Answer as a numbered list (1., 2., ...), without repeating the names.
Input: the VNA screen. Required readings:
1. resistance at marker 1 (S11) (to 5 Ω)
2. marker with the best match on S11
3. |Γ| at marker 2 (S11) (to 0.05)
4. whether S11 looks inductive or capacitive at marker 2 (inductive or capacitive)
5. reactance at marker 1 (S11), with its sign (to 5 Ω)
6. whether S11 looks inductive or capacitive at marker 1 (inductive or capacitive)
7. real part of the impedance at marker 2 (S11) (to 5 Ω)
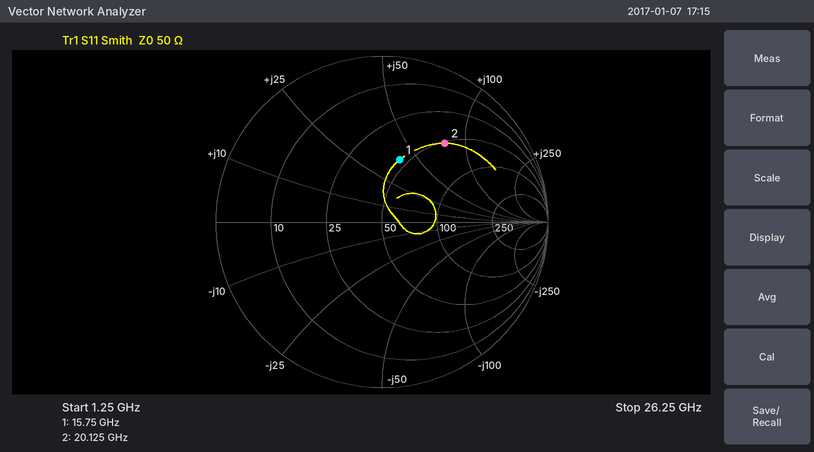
1. 45 Ω
2. marker 1
3. 0.60
4. inductive
5. +40 Ω
6. inductive
7. 50 Ω
